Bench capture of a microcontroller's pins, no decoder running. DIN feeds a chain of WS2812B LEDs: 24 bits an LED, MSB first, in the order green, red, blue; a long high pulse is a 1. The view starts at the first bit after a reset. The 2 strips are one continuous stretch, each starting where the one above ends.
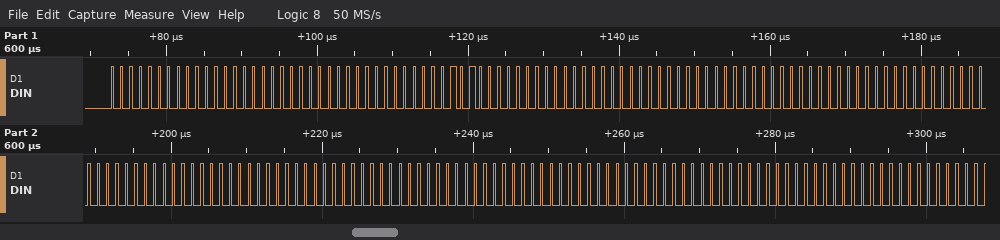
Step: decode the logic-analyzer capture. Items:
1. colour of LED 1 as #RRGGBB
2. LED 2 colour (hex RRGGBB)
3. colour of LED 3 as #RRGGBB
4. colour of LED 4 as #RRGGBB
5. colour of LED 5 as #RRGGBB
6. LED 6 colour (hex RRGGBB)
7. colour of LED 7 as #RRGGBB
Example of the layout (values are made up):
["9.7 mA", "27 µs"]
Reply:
["#000000", "#0A0000", "#000000", "#000000", "#000000", "#000000", "#000000"]
